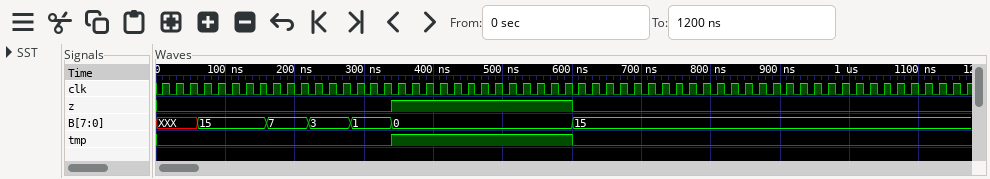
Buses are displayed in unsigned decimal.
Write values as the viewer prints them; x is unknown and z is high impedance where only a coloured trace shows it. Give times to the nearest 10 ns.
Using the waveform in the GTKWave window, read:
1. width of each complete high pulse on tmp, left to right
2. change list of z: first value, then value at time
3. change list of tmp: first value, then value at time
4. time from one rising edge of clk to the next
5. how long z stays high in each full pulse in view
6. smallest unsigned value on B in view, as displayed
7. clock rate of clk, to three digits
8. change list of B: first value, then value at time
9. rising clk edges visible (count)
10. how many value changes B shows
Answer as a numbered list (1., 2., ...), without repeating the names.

1. 260 ns
2. 0, 1 at 340 ns, 0 at 600 ns
3. 0, 1 at 340 ns, 0 at 600 ns
4. 20 ns
5. 260 ns
6. 0
7. 50.0 MHz
8. XXX, 15 at 60 ns, 7 at 160 ns, 3 at 220 ns, 1 at 280 ns, 0 at 340 ns, 15 at 600 ns
9. 59
10. 6
